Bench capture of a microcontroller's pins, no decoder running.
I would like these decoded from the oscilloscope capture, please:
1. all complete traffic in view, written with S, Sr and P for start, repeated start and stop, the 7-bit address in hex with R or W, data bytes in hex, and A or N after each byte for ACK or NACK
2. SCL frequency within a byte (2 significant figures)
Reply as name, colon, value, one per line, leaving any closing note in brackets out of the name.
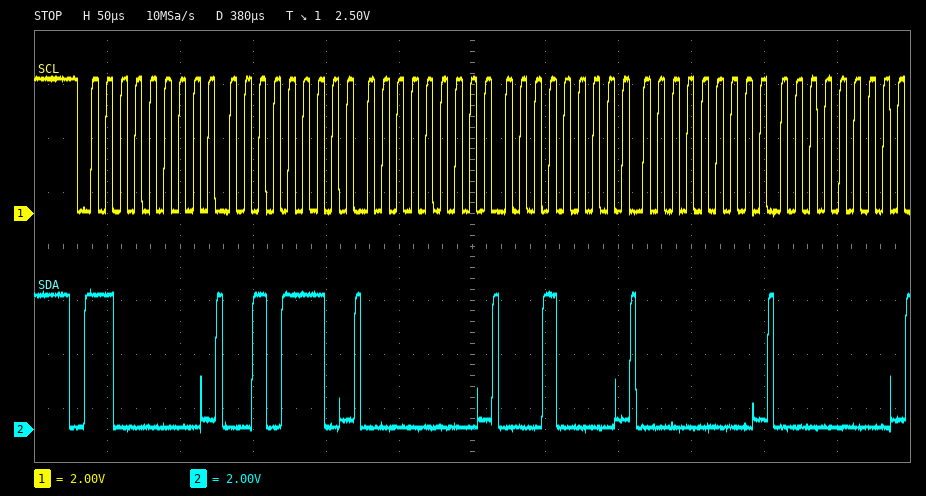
all complete traffic in view, written with S, Sr and P for start, repeated start and stop, the 7-bit address in hex with R or W, data bytes in hex, and A or N after each byte for ACK or NACK: S 60W A 2E A 00 A 10 A 00 A 00 A
SCL frequency within a byte: 100 kHz
